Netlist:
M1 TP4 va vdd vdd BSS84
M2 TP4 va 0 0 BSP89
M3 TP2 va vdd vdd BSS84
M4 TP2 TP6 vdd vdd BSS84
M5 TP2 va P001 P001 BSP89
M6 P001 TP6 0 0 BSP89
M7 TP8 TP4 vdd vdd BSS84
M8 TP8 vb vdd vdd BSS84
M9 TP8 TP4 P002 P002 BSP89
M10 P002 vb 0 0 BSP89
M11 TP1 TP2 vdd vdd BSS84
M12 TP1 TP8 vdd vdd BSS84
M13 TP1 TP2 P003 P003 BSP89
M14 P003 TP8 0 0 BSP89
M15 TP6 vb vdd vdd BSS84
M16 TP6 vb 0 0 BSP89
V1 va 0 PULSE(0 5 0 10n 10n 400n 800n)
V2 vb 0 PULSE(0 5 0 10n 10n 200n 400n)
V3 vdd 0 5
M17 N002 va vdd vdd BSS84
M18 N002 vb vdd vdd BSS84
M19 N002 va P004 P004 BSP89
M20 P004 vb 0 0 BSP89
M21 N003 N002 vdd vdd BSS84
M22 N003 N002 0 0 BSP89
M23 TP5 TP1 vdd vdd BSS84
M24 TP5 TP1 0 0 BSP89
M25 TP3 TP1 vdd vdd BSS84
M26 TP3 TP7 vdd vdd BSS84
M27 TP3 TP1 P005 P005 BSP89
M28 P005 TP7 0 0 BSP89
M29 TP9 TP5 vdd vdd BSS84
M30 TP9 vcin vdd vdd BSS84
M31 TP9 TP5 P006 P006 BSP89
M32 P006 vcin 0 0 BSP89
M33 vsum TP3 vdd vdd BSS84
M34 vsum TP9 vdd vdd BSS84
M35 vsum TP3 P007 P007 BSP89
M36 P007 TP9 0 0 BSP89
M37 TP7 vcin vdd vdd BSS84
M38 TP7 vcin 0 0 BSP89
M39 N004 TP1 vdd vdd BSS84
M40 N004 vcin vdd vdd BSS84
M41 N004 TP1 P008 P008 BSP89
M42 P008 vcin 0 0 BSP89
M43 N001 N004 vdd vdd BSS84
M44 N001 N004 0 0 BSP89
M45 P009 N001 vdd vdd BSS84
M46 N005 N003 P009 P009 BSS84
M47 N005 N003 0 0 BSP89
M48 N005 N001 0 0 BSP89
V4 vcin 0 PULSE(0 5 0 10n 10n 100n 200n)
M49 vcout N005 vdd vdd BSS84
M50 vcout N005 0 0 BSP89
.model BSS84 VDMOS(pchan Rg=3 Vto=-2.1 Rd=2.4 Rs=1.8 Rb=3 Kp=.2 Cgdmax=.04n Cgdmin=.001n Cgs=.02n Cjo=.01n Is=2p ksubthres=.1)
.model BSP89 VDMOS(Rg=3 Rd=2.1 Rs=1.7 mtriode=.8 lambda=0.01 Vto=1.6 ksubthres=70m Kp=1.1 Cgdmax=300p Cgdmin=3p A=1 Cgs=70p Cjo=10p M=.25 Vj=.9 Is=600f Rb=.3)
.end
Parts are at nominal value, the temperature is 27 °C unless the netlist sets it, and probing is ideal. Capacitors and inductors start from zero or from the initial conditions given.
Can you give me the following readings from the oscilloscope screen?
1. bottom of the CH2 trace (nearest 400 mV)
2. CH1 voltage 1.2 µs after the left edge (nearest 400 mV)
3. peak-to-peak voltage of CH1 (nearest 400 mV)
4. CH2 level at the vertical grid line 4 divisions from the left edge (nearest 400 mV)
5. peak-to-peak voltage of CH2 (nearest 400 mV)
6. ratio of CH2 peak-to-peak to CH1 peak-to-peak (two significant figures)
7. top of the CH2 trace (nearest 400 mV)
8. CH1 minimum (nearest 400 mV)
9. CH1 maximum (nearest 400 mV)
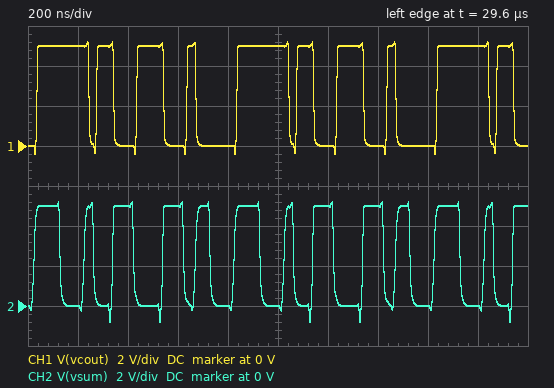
-800 mV
0 V
5.6 V
0 V
6.0 V
1.1
5.2 V
-400 mV
5.2 V
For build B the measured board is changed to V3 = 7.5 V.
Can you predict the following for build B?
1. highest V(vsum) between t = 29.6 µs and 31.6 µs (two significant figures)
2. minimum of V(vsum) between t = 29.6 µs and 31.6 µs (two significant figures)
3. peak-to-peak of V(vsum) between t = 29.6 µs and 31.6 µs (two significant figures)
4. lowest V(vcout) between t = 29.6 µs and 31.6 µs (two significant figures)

7.7 V
-1.0 V
8.7 V
-490 mV
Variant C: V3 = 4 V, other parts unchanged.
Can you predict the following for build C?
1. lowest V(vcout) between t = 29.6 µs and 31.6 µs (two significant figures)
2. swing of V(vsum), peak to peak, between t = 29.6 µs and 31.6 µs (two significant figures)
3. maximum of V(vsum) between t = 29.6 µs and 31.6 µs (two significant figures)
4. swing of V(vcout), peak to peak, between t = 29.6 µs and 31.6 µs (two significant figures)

-360 mV
5.0 V
4.3 V
4.6 V
